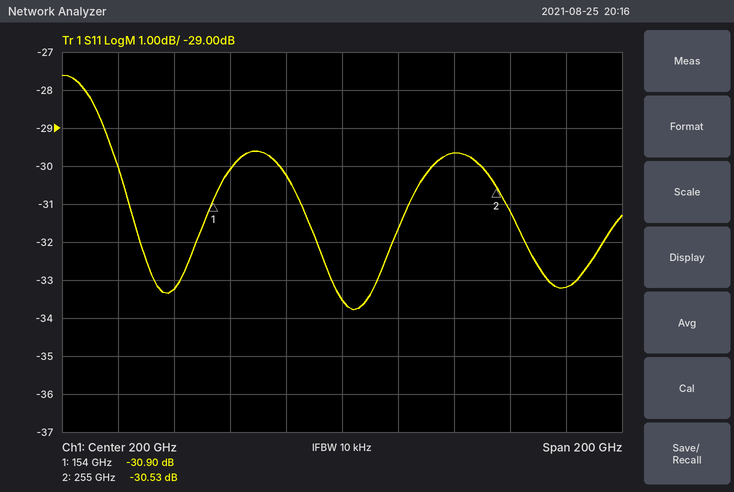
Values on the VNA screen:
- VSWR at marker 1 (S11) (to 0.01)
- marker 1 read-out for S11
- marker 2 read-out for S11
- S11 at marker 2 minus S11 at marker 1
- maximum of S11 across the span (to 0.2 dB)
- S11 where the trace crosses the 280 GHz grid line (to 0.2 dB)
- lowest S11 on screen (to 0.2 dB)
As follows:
1.06
-30.90 dB
-30.53 dB
0.37 dB
-27.6 dB
-33.2 dB
-33.8 dB
